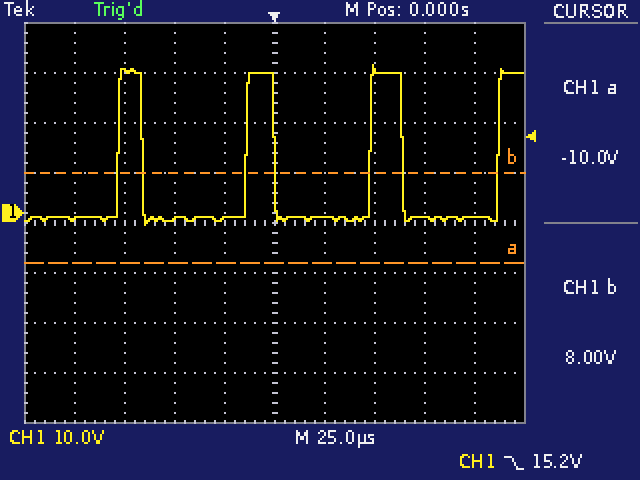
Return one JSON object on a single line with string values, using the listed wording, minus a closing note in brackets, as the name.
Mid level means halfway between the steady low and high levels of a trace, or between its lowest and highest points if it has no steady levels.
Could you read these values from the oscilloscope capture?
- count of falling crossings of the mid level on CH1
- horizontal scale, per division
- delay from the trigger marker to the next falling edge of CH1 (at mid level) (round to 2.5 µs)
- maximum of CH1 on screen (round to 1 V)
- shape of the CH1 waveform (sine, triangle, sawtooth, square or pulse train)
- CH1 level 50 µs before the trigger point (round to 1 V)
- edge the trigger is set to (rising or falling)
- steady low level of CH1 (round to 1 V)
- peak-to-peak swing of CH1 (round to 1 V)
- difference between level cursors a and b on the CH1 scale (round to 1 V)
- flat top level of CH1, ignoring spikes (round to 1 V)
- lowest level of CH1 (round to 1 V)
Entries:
{"count of falling crossings of the mid level on CH1": "3", "horizontal scale, per division": "25 µs", "delay from the trigger marker to the next falling edge of CH1 (at mid level)": "65.0 µs", "maximum of CH1 on screen": "30 V", "shape of the CH1 waveform": "pulse train", "CH1 level 50 µs before the trigger point": "-1 V", "edge the trigger is set to": "falling", "steady low level of CH1": "-1 V", "peak-to-peak swing of CH1": "32 V", "difference between level cursors a and b on the CH1 scale": "18 V", "flat top level of CH1, ignoring spikes": "28 V", "lowest level of CH1": "-2 V"}
